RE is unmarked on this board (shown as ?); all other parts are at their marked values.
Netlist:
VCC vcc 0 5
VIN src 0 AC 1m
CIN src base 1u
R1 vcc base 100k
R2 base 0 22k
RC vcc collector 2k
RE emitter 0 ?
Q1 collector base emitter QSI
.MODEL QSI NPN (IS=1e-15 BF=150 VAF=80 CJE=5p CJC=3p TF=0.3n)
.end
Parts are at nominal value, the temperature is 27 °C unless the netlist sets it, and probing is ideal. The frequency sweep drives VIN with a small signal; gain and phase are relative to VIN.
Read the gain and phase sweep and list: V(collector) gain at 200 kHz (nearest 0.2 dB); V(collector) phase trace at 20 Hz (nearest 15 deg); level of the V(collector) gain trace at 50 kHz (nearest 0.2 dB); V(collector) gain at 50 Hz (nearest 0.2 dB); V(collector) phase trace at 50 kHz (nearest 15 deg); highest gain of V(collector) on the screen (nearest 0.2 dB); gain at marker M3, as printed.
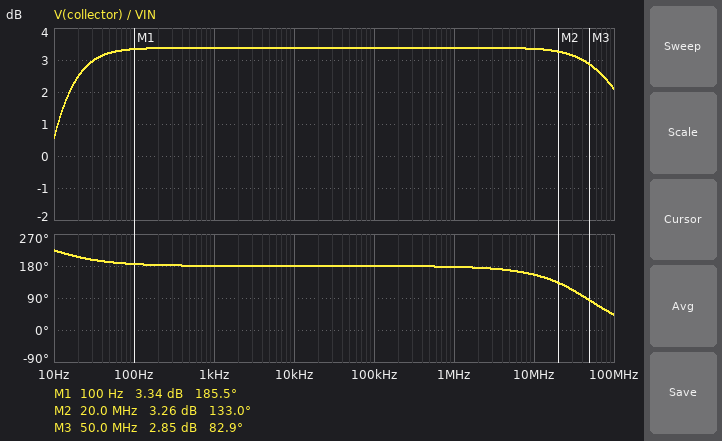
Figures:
3.4 dB
210 deg
3.4 dB
3.2 dB
180 deg
3.4 dB
2.85 dB
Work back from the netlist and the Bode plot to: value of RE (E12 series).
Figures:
1.2 kΩ
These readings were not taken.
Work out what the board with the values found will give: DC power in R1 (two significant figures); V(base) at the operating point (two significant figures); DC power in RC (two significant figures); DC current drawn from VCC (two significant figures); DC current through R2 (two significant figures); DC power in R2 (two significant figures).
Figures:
170 µW
880 mV
62 µW
220 µA
40 µA
35 µW
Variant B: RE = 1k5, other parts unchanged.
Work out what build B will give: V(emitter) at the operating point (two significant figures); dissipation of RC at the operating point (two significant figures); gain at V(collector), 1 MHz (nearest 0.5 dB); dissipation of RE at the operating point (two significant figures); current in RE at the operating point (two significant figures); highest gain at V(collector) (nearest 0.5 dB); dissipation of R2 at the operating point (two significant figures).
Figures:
220 mV
43 µW
1.5 dB
33 µW
150 µA
2.0 dB
36 µW
